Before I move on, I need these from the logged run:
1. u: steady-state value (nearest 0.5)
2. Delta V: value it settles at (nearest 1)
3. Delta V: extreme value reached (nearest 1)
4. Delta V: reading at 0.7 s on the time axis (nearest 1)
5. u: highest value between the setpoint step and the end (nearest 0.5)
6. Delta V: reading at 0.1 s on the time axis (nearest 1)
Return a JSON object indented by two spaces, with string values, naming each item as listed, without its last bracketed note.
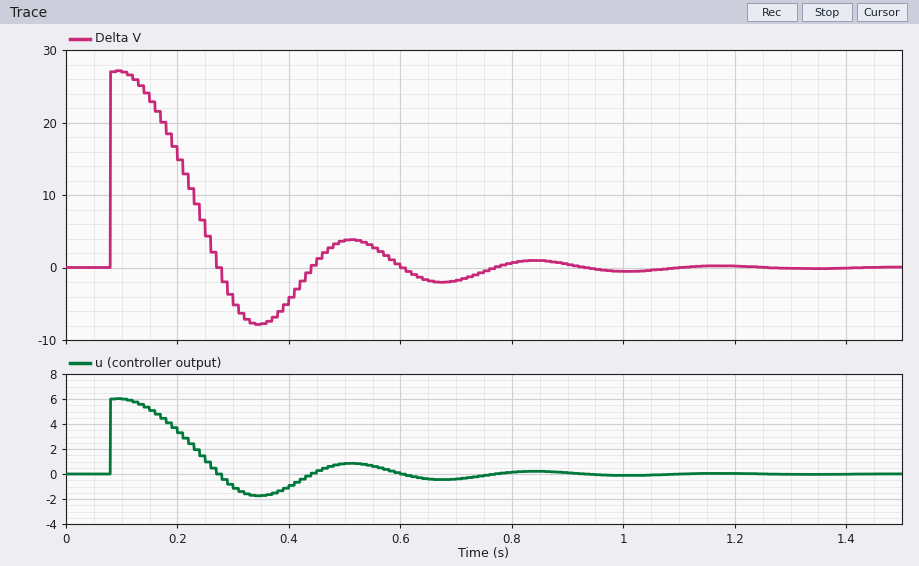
{
  "u: steady-state value": "0.0",
  "Delta V: value it settles at": "0",
  "Delta V: extreme value reached": "27",
  "Delta V: reading at 0.7 s on the time axis": "-2",
  "u: highest value between the setpoint step and the end": "6.0",
  "Delta V: reading at 0.1 s on the time axis": "27"
}
